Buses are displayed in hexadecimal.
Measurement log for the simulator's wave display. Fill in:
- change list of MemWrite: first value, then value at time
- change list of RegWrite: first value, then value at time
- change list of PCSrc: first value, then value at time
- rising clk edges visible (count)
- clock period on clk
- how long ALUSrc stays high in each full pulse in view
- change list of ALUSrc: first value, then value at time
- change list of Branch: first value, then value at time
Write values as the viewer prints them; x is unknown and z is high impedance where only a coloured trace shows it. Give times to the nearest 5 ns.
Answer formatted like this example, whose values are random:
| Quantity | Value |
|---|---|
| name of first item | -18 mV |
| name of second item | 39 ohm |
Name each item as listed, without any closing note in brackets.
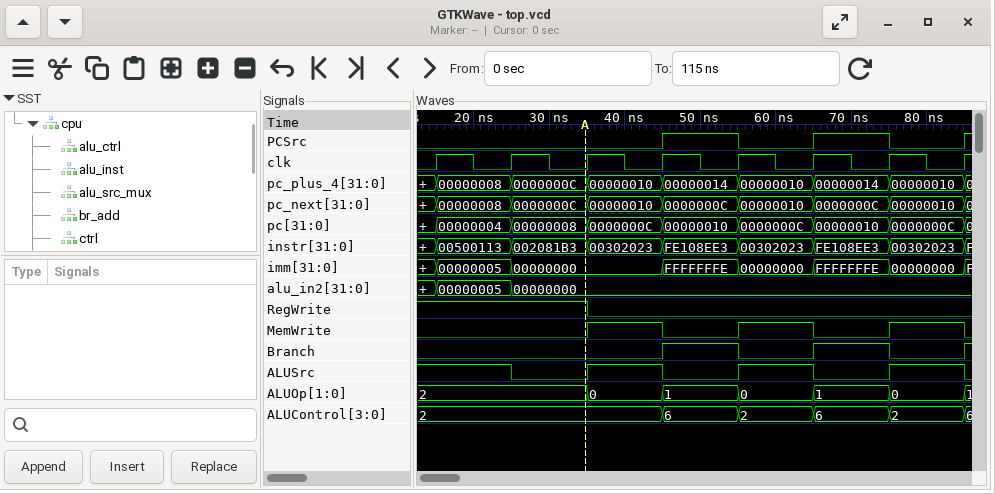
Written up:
| Quantity | Value |
|---|---|
| change list of MemWrite: first value, then value at time | 0, 1 at 35 ns, 0 at 45 ns, 1 at 55 ns, 0 at 65 ns, 1 at 75 ns, 0 at 85 ns |
| change list of RegWrite: first value, then value at time | 1, 0 at 35 ns |
| change list of PCSrc: first value, then value at time | 0, 1 at 45 ns, 0 at 55 ns, 1 at 65 ns, 0 at 75 ns, 1 at 85 ns |
| rising clk edges visible | 8 |
| clock period on clk | 10 ns |
| how long ALUSrc stays high in each full pulse in view | 10 ns, 10 ns, 10 ns |
| change list of ALUSrc: first value, then value at time | 1, 0 at 25 ns, 1 at 35 ns, 0 at 45 ns, 1 at 55 ns, 0 at 65 ns, 1 at 75 ns, 0 at 85 ns |
| change list of Branch: first value, then value at time | 0, 1 at 45 ns, 0 at 55 ns, 1 at 65 ns, 0 at 75 ns, 1 at 85 ns |
